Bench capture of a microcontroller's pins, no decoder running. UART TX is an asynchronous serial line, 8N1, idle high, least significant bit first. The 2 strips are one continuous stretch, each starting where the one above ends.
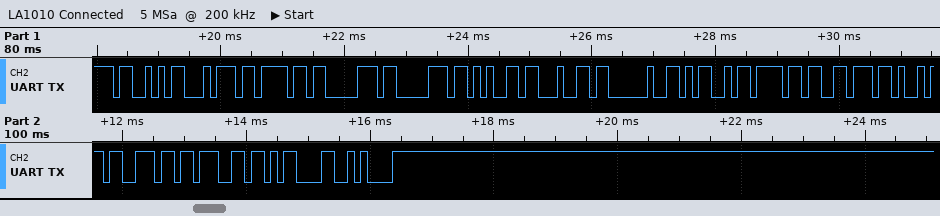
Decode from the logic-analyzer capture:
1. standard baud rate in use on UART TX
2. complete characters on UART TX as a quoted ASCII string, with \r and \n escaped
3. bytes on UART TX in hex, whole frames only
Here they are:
9600 baud
"Stopped Moving\r\n"
53 74 6F 70 70 65 64 20 4D 6F 76 69 6E 67 0D 0A
